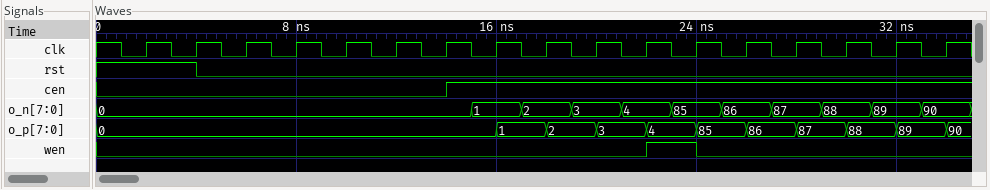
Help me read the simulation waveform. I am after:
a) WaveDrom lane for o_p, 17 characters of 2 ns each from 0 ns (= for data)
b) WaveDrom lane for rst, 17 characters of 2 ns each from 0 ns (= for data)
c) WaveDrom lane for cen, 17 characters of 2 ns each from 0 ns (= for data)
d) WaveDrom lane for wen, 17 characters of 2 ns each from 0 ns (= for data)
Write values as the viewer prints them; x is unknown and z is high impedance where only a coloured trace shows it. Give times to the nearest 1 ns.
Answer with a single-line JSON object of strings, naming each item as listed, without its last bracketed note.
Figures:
{"WaveDrom lane for o_p, 17 characters of 2 ns each from 0 ns": "{name: 'o_p', wave: '=.......=========', data: '0 1 2 3 4 85 86 87 88 89'}", "WaveDrom lane for rst, 17 characters of 2 ns each from 0 ns": "{name: 'rst', wave: '1.0..............'}", "WaveDrom lane for cen, 17 characters of 2 ns each from 0 ns": "{name: 'cen', wave: '0......1.........'}", "WaveDrom lane for wen, 17 characters of 2 ns each from 0 ns": "{name: 'wen', wave: '0..........10....'}"}
